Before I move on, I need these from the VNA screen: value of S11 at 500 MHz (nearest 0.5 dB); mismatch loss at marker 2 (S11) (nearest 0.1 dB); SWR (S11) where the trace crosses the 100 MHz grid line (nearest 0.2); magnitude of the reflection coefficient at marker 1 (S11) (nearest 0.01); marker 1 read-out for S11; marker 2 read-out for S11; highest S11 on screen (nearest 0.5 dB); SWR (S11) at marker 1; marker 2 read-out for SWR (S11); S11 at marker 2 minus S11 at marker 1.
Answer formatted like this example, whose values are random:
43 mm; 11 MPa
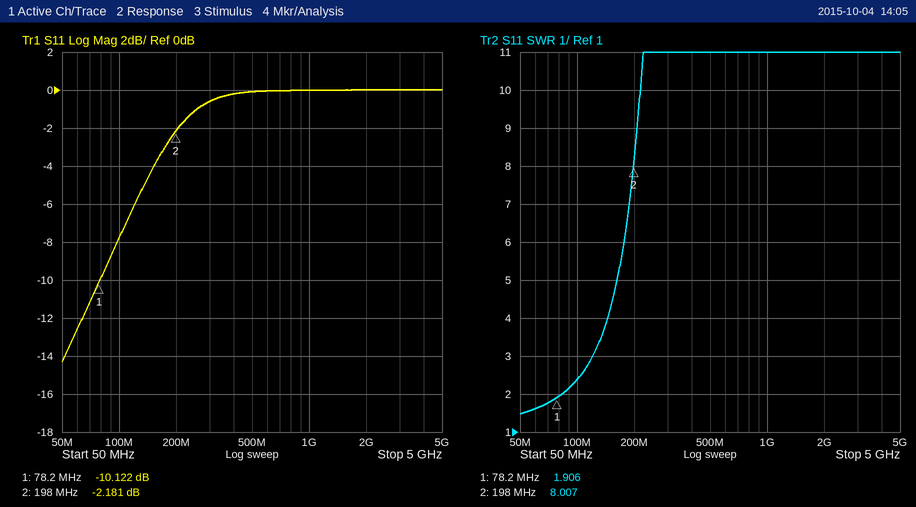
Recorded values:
0.0 dB; 4.0 dB; 2.4; 0.31; -10.122 dB; -2.181 dB; 0.0 dB; 1.906; 8.007; 7.941 dB
